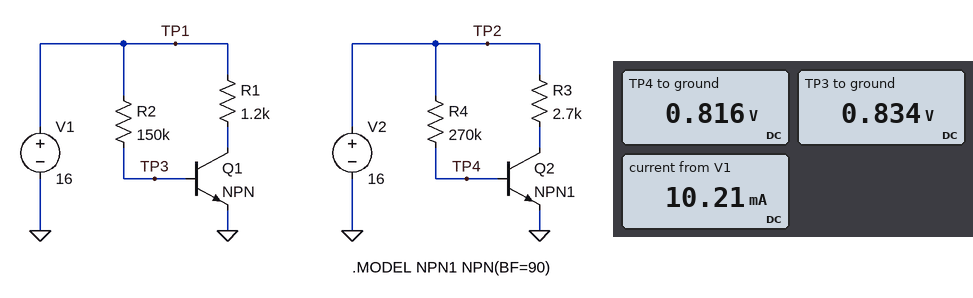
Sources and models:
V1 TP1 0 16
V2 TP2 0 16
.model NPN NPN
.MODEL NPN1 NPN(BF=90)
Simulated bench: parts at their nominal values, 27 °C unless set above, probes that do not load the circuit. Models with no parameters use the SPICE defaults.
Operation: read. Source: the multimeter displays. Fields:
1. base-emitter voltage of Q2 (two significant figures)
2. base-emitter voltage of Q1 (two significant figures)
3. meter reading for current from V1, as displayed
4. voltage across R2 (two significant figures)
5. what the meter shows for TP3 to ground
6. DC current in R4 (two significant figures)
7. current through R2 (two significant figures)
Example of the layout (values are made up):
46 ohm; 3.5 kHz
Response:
820 mV; 830 mV; 10.21 mA; 15 V; 0.834 V; 56 µA; 100 µA
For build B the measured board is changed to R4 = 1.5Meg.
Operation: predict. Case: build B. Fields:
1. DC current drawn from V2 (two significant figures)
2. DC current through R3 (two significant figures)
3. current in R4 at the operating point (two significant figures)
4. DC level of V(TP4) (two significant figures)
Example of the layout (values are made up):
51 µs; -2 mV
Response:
920 µA; 910 µA; 10 µA; 770 mV
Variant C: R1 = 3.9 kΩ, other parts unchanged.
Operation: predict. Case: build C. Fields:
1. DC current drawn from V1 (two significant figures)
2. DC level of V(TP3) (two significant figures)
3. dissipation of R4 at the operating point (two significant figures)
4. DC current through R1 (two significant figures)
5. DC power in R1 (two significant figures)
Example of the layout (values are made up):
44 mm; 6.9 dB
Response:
4.2 mA; 810 mV; 850 µW; 4.1 mA; 65 mW
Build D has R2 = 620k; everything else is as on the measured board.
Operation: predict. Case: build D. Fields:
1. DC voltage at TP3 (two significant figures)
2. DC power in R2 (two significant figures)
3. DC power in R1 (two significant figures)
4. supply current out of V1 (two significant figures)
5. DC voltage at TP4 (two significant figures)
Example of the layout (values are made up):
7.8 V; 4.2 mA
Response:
800 mV; 370 µW; 7.2 mW; 2.5 mA; 820 mV
